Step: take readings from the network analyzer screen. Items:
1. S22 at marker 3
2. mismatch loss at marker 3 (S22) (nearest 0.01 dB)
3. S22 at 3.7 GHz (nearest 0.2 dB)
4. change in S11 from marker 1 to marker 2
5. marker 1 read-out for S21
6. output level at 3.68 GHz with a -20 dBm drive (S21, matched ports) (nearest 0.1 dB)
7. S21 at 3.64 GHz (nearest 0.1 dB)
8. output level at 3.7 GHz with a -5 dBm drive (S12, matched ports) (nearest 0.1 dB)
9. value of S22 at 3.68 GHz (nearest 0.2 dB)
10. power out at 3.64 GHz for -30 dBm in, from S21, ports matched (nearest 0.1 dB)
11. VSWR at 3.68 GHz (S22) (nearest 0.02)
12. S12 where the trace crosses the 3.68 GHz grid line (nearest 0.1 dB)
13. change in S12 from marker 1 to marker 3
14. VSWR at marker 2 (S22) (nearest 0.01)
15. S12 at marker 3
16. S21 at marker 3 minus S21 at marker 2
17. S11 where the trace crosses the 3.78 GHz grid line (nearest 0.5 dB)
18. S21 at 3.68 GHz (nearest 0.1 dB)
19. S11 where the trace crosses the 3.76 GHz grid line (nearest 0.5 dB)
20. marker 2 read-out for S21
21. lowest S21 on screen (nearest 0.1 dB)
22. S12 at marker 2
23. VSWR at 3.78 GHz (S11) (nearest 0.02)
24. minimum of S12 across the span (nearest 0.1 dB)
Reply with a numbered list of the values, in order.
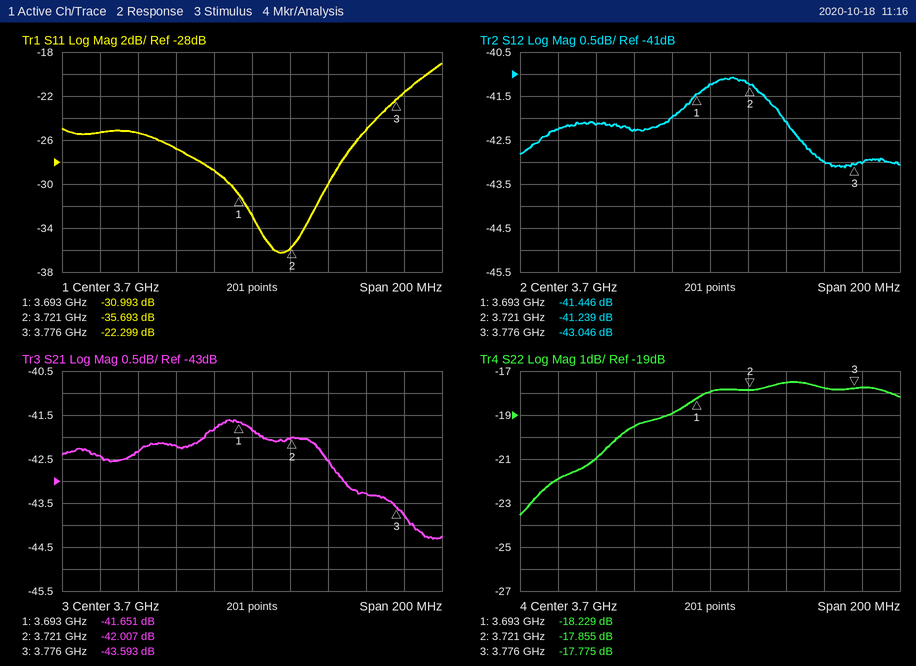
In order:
1. -17.775 dB
2. 0.07 dB
3. -18.0 dB
4. -4.700 dB
5. -41.651 dB
6. -61.8 dBm
7. -42.3 dB
8. -46.2 dBm
9. -19.0 dB
10. -72.3 dBm
11. 1.26
12. -42.0 dB
13. -1.600 dB
14. 1.29
15. -43.046 dB
16. -1.586 dB
17. -21.5 dB
18. -41.8 dB
19. -25.0 dB
20. -42.007 dB
21. -44.3 dB
22. -41.239 dB
23. 1.18
24. -43.1 dB
